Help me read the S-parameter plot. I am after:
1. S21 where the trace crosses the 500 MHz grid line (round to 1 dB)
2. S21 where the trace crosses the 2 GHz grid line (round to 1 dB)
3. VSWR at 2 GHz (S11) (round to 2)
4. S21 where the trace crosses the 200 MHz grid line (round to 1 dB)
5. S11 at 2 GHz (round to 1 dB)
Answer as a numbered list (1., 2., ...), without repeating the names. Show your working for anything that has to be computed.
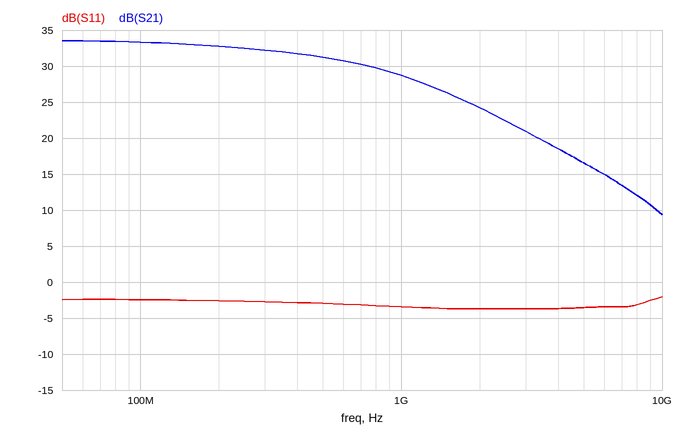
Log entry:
1. 31 dB
2. 24 dB
3. |Γ| = 10^(-4/20) = 0.6310; VSWR = (1 + 0.6310)/(1 − 0.6310) ≈ 4
4. 33 dB
5. -4 dB
